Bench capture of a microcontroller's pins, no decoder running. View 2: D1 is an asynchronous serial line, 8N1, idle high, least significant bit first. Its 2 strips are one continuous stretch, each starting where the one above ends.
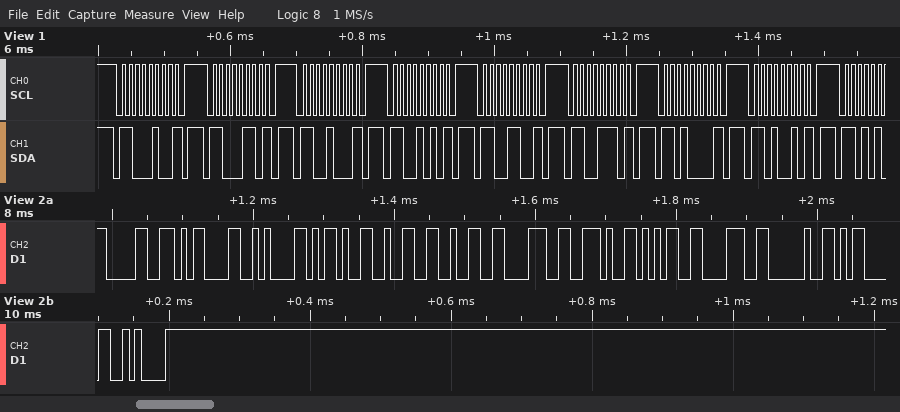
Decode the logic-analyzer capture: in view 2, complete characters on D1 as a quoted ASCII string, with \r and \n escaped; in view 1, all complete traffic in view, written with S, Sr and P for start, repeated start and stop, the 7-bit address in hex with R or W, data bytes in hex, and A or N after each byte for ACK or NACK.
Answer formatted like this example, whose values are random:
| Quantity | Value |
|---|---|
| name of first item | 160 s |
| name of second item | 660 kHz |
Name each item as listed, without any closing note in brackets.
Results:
| Quantity | Value |
|---|---|
| in view 2, complete characters on D1 as a quoted ASCII string, with \r and \n escaped | "0\r\n-228.58 \r\n" |
| in view 1, all complete traffic in view, written with S, Sr and P for start, repeated start and stop, the 7-bit address in hex with R or W, data bytes in hex, and A or N after each byte for ACK or NACK | S 62W N P S 63W N P S 64W N P S 65W N P S 66W N P S 67W N P S 68W N P S 69W N P |
